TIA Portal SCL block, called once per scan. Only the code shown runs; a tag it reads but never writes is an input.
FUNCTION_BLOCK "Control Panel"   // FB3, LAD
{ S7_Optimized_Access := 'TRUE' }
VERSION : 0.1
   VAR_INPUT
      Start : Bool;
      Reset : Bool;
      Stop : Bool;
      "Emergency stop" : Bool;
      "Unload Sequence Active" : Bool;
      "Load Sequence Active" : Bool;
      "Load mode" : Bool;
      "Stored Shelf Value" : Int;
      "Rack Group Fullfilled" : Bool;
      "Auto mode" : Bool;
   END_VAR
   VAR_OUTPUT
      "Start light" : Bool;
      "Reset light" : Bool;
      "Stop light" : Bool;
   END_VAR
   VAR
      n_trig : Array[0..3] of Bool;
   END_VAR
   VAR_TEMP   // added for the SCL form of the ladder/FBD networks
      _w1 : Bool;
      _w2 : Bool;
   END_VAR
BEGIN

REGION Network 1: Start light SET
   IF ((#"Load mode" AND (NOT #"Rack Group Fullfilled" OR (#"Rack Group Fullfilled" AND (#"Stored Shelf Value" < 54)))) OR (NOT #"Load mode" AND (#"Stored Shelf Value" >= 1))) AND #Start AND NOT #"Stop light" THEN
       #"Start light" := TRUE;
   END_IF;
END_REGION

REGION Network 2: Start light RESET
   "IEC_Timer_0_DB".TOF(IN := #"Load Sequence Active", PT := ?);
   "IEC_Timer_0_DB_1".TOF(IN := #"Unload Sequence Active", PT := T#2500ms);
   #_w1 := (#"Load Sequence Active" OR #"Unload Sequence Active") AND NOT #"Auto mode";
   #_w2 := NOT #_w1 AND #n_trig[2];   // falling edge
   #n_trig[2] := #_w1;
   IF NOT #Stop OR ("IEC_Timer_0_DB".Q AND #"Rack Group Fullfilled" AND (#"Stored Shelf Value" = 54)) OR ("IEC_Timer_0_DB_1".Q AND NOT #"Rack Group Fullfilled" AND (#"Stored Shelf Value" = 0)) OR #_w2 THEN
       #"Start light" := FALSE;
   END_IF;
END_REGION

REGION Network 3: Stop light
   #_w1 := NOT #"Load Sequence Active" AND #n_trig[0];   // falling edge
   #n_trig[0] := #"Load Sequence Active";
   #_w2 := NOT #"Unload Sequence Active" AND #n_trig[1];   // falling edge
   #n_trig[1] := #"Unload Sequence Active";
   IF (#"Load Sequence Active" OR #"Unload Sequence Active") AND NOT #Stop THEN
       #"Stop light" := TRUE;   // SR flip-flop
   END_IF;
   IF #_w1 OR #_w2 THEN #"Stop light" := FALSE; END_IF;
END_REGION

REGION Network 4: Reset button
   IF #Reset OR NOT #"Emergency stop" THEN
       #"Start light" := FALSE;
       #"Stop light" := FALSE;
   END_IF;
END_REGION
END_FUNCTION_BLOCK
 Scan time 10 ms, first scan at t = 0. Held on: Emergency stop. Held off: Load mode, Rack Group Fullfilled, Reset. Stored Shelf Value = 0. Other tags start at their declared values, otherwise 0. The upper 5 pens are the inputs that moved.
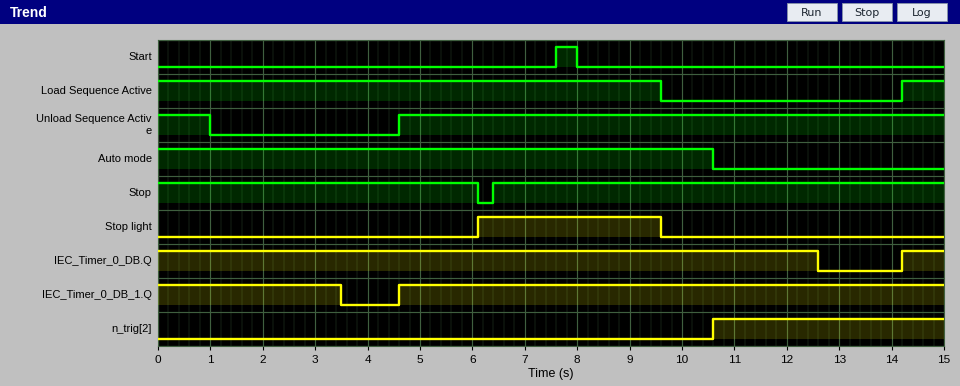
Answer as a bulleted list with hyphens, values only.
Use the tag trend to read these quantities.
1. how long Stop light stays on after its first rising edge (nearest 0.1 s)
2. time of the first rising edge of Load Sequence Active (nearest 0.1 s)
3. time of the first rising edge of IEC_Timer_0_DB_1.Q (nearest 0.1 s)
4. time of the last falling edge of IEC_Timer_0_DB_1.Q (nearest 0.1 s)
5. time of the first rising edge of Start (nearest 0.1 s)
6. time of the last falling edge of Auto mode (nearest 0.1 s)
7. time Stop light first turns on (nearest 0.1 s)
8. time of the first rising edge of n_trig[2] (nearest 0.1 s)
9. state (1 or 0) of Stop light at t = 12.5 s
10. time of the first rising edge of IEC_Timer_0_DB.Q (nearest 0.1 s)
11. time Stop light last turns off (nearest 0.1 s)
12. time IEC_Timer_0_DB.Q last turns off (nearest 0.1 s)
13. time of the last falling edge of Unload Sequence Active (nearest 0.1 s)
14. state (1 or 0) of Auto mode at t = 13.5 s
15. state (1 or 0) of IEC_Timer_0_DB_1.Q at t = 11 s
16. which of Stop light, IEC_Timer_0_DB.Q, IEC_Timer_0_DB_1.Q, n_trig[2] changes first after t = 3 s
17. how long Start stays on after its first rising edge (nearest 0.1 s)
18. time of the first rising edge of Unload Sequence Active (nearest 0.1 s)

- 3.5 s
- 14.2 s
- 4.6 s
- 3.5 s
- 7.6 s
- 10.6 s
- 6.1 s
- 10.6 s
- 0
- 14.2 s
- 9.6 s
- 12.6 s
- 1.0 s
- 0
- 1
- IEC_Timer_0_DB_1.Q
- 0.4 s
- 4.6 s
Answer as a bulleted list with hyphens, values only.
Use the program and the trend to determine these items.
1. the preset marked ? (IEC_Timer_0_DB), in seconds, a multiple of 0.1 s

- 3.0 s
